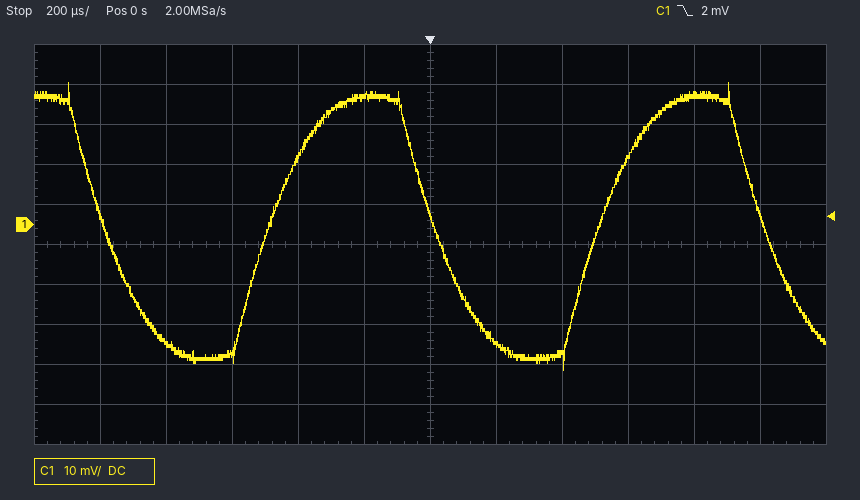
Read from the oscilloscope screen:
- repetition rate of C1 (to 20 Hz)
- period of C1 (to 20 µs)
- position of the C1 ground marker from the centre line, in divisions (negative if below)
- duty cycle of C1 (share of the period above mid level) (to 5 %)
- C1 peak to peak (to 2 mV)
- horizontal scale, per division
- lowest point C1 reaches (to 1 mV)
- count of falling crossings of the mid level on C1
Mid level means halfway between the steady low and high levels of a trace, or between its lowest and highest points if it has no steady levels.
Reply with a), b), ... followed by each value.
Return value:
a) 1.00 kHz
b) 1.00 ms
c) +0.5 div
d) 50 %
e) 72 mV
f) 200 µs
g) -36 mV
h) 3
